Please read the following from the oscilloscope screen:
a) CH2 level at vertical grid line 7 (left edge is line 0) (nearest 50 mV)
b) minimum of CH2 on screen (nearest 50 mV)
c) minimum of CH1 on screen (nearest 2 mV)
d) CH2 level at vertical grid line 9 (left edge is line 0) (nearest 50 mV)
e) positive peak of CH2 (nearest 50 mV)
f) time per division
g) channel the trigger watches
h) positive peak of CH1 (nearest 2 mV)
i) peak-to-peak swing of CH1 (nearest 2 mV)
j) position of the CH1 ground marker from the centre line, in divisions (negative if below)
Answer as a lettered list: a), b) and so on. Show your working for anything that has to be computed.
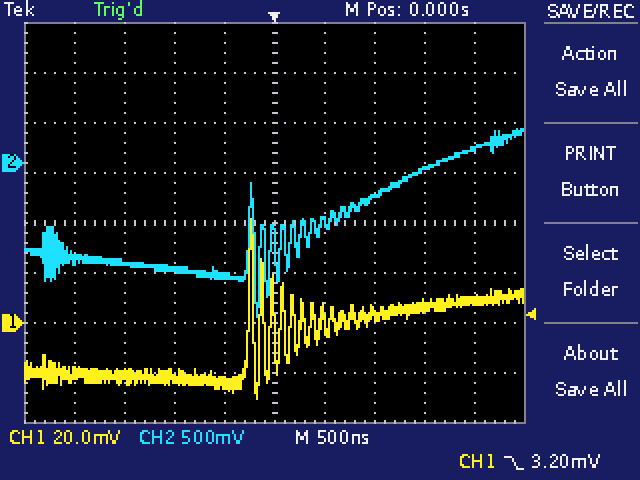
a) -350 mV
b) -1.55 V
c) -30 mV
d) 150 mV
e) 350 mV
f) 500 ns
g) CH1
h) 42 mV
i) 42 mV − (-30 mV) = 72 mV
j) -2.0 div
